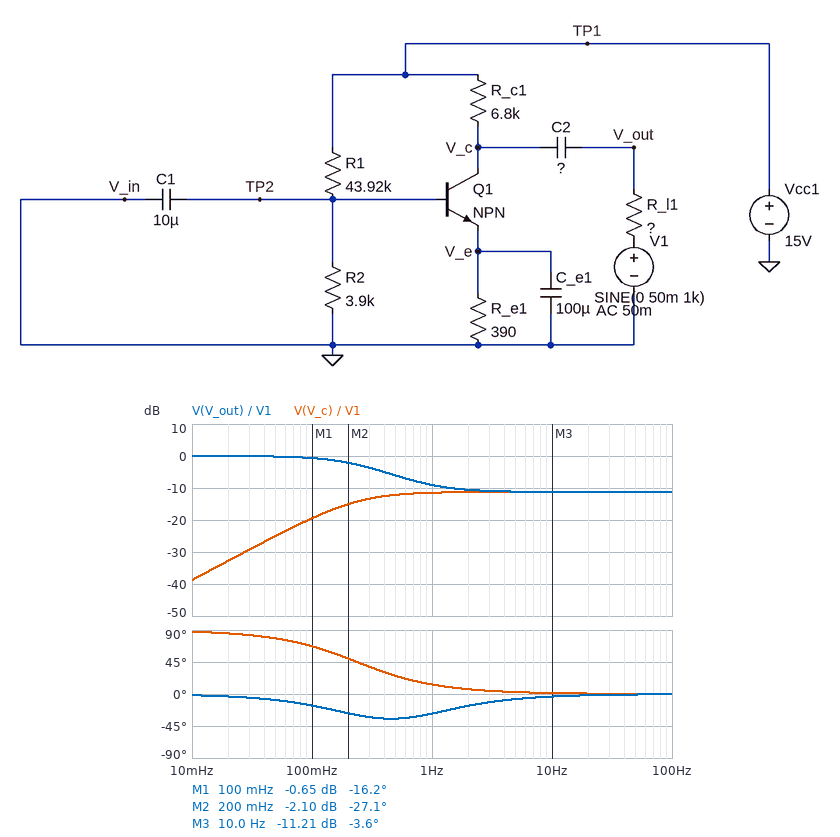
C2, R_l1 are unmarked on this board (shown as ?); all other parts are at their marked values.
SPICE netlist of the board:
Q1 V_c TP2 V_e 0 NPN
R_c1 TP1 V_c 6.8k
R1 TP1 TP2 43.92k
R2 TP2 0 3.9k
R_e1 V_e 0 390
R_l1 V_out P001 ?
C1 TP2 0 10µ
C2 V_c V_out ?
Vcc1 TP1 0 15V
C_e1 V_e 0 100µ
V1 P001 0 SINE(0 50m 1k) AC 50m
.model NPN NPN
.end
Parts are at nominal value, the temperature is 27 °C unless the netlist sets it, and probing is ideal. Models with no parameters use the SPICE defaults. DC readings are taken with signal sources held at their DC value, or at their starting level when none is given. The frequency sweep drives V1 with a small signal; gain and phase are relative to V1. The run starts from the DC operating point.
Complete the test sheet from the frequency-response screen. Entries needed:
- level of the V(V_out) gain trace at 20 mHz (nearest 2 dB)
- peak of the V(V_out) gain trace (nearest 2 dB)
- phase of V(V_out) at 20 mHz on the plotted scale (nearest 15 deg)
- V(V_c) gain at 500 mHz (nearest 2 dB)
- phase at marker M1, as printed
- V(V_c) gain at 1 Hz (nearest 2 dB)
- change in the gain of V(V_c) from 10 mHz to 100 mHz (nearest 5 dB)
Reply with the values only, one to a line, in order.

0 dB
0 dB
0 deg
-12 dB
-16.2 deg
-12 dB
20 dB
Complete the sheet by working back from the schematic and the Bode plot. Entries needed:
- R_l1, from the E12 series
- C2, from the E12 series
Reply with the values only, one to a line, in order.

18 kΩ
27 µF
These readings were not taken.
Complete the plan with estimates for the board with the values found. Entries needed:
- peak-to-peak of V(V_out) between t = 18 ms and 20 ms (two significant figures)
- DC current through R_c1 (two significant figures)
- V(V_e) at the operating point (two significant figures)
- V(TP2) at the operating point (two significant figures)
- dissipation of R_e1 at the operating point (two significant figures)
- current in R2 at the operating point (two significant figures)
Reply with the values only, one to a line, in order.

27 mV
1.0 mA
410 mV
1.2 V
430 µW
300 µA
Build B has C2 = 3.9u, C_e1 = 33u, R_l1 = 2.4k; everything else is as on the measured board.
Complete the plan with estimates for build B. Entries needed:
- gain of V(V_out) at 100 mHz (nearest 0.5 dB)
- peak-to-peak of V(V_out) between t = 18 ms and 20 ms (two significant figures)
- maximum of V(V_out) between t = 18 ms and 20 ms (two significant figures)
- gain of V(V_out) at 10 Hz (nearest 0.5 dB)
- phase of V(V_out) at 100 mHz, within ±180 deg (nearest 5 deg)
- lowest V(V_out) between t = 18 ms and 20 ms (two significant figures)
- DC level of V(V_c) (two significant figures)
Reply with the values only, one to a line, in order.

0 dB
74 mV
37 mV
-2.0 dB
0 deg
-37 mV
7.9 V
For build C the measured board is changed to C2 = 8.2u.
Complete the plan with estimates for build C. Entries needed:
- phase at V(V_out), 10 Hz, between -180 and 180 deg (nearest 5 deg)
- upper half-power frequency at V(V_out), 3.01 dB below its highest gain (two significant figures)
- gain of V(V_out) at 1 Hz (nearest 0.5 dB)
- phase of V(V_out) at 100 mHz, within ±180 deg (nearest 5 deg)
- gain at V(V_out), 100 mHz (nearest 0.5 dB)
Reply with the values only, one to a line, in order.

-10 deg
850 mHz
-3.5 dB
-5 deg
0 dB
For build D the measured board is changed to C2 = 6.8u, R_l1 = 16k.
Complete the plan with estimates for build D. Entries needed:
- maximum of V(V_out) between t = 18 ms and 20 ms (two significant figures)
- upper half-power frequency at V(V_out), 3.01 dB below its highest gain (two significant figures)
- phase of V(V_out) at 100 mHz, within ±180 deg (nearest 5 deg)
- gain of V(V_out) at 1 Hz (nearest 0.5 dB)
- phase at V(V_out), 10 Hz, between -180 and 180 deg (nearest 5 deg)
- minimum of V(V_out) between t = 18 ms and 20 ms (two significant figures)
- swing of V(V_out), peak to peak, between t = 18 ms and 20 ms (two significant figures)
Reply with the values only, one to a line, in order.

15 mV
1.1 Hz
-5 deg
-2.5 dB
-15 deg
-15 mV
30 mV
